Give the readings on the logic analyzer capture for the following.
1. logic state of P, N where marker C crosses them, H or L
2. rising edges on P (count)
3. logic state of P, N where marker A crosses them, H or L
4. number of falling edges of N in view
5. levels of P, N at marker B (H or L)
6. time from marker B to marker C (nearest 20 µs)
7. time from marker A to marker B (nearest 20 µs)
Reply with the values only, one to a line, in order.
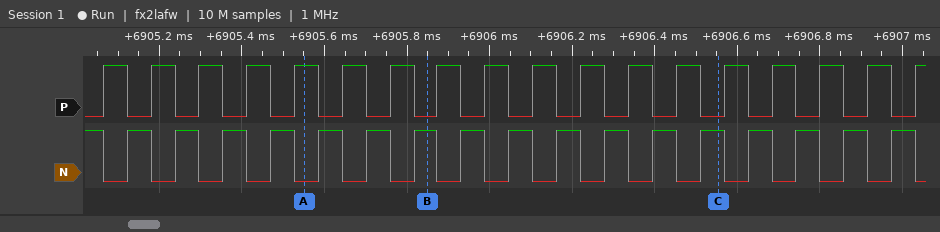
P=L, N=H
18
P=H, N=L
18
P=L, N=H
700 µs
300 µs
